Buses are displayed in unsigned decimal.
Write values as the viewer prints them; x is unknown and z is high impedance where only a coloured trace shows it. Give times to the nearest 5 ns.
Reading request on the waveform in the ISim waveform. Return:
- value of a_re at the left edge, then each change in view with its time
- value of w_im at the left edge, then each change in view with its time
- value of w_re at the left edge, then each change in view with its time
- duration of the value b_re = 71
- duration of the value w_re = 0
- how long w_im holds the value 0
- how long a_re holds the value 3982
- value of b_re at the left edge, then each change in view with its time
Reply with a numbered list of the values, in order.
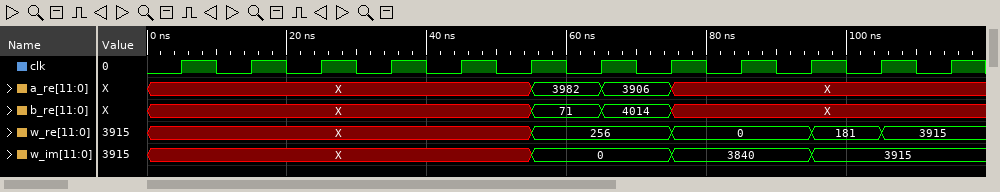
1. X, 3982 at 55 ns, 3906 at 65 ns, X at 75 ns
2. X, 0 at 55 ns, 3840 at 75 ns, 3915 at 95 ns
3. X, 256 at 55 ns, 0 at 75 ns, 181 at 95 ns, 3915 at 105 ns
4. 10 ns
5. 20 ns
6. 20 ns
7. 10 ns
8. X, 71 at 55 ns, 4014 at 65 ns, X at 75 ns
